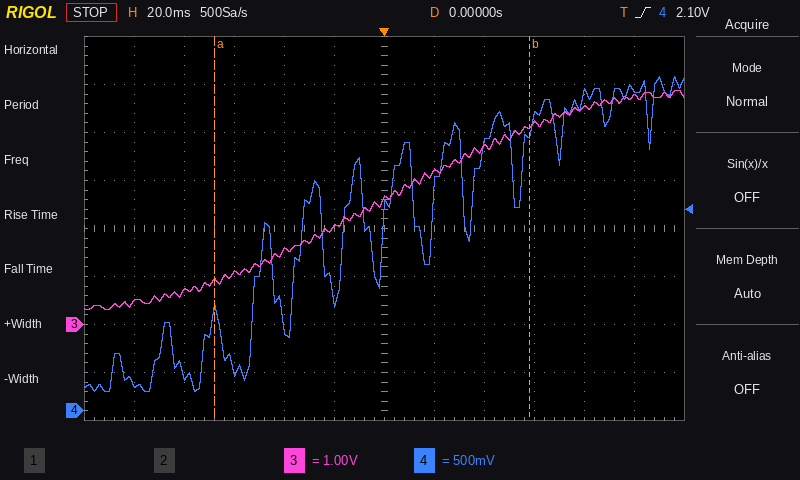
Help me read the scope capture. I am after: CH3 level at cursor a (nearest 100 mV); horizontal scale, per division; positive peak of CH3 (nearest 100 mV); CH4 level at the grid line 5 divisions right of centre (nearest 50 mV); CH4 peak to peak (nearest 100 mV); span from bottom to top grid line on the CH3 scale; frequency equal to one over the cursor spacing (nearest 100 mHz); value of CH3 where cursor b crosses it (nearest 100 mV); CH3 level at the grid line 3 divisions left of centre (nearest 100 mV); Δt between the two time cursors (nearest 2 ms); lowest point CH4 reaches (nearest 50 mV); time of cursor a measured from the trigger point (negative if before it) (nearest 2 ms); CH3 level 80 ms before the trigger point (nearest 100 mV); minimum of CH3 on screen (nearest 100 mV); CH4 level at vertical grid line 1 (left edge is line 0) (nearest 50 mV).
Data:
900 mV
20 ms
4.9 V
3.35 V
3.30 V
8 V
7.9 Hz
4.1 V
1.1 V
126 ms
200 mV
-68 ms
700 mV
300 mV
300 mV
